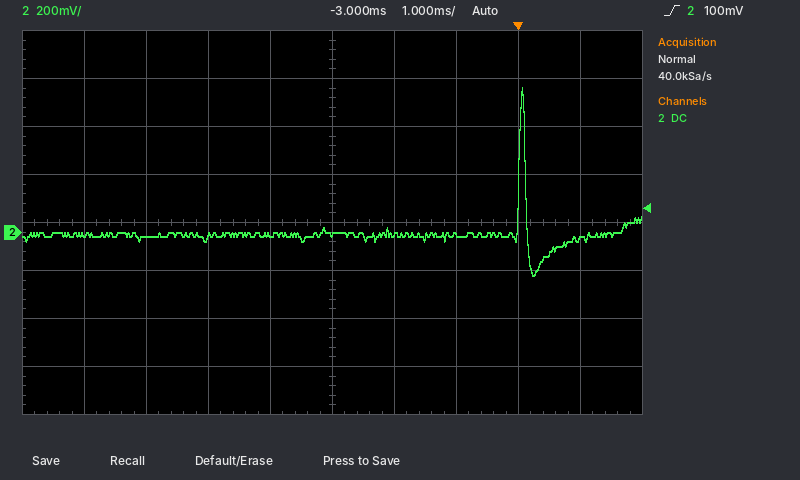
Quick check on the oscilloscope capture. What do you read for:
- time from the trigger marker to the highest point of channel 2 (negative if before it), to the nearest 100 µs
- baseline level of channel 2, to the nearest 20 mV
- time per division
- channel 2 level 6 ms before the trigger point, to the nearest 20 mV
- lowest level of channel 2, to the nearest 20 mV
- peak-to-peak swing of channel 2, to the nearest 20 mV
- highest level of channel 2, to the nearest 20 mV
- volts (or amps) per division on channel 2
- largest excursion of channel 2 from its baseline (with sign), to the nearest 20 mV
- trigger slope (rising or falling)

+100 µs
-20 mV
1 ms
-20 mV
-180 mV
780 mV
600 mV
200 mV
+620 mV
rising
